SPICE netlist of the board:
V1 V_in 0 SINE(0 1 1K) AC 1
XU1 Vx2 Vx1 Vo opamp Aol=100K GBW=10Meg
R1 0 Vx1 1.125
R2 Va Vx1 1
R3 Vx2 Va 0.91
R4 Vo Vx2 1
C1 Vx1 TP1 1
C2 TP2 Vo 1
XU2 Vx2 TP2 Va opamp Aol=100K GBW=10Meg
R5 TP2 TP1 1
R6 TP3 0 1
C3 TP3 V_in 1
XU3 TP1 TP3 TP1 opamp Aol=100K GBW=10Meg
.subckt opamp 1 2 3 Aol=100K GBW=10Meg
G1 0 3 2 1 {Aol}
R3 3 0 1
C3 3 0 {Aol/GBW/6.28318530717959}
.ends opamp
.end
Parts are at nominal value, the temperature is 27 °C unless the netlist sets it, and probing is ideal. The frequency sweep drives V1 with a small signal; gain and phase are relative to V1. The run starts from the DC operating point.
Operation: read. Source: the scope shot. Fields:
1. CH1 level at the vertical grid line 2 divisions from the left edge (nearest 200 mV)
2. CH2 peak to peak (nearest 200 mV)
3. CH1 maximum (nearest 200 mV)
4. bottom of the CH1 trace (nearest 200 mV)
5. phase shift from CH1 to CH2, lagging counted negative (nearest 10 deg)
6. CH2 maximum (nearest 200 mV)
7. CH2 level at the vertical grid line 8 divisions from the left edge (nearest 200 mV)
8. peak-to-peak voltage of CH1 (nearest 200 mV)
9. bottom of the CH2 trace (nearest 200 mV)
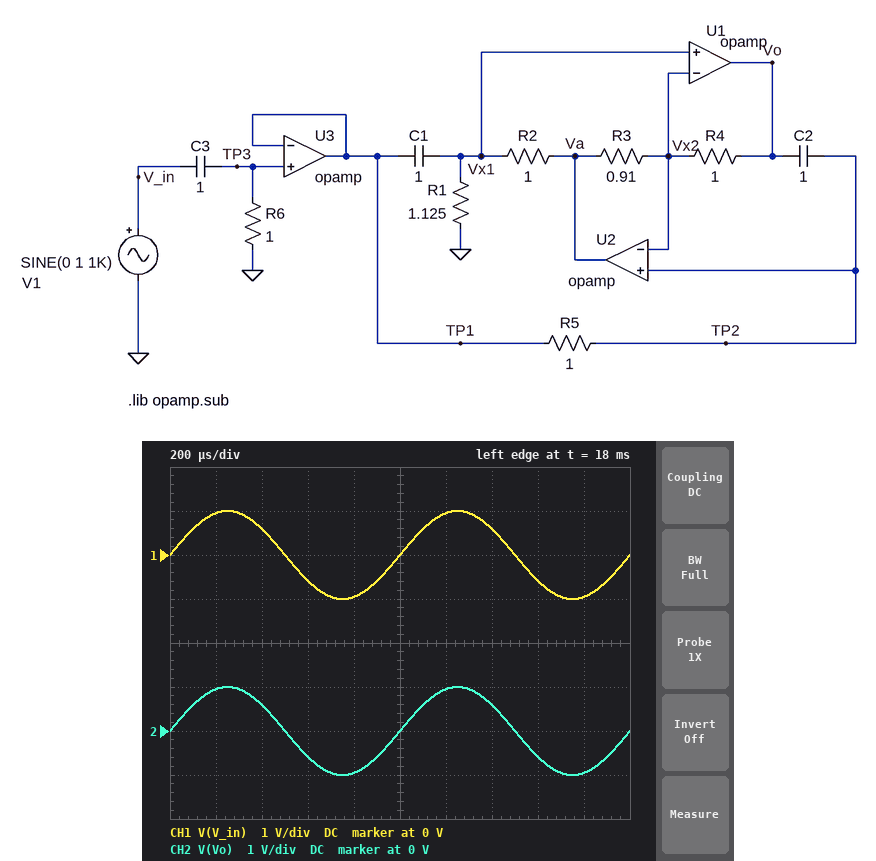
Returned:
600 mV
2.0 V
1.0 V
-1.0 V
0 deg
1.0 V
-600 mV
2.0 V
-1.0 V
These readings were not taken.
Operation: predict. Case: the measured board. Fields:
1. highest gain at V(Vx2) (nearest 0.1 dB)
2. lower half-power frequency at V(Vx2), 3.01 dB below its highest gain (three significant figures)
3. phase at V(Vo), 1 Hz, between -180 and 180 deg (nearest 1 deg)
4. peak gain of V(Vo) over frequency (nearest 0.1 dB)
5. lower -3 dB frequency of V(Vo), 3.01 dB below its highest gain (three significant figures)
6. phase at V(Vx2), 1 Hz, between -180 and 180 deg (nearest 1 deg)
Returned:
0 dB
280 mHz
17 deg
0 dB
150 mHz
17 deg
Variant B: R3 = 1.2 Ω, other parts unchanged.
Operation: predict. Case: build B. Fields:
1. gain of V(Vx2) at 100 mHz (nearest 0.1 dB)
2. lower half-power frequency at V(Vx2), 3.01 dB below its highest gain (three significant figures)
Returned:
-7.2 dB
294 mHz
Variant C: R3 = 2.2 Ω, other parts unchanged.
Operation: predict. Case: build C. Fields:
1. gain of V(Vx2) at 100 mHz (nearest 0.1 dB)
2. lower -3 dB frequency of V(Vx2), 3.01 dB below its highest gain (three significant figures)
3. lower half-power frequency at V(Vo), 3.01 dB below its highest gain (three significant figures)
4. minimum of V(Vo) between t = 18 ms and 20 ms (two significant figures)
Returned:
-5.9 dB
340 mHz
253 mHz
-1.0 V
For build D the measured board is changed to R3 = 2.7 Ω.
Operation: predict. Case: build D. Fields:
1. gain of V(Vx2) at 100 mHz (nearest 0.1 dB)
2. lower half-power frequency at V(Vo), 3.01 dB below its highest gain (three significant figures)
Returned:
-5.7 dB
282 mHz
